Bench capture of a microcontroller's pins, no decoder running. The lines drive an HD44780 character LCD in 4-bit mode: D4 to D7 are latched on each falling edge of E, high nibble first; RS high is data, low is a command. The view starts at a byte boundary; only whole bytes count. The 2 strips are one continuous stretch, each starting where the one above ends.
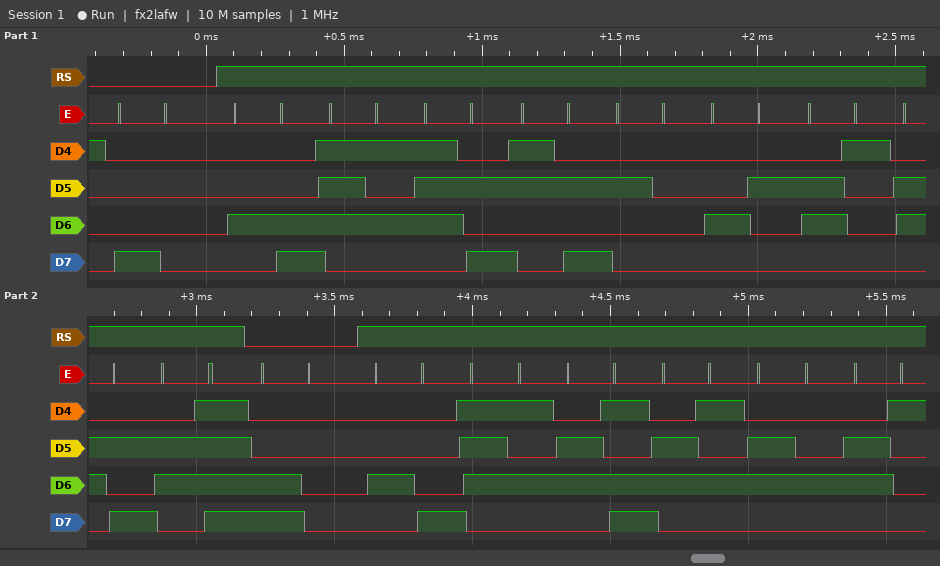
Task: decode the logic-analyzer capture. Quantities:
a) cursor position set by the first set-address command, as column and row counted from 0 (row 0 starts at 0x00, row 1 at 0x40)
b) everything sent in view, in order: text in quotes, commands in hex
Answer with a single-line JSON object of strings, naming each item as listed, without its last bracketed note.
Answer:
{"cursor position set by the first set-address command, as column and row counted from 0": "column 0, row 0", "everything sent in view, in order: text in quotes, commands in hex": "0x80 \"Luz: Bajo\" 0xC0 \"Humeda\""}
